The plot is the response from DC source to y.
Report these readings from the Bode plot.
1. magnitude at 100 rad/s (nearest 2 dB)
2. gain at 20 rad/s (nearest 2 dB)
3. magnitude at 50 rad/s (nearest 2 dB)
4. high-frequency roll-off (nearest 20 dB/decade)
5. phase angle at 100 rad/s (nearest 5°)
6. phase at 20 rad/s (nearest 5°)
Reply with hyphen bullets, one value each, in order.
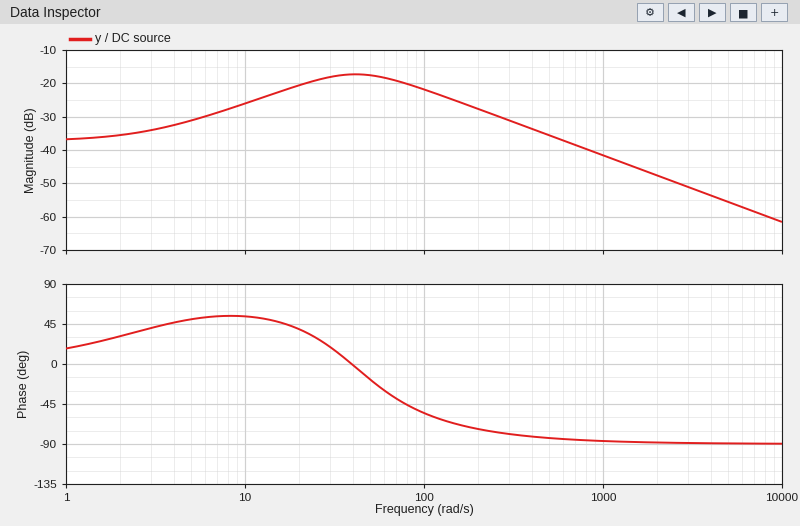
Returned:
- -22 dB
- -20 dB
- -18 dB
- -20 dB/decade
- -55°
- 40°
